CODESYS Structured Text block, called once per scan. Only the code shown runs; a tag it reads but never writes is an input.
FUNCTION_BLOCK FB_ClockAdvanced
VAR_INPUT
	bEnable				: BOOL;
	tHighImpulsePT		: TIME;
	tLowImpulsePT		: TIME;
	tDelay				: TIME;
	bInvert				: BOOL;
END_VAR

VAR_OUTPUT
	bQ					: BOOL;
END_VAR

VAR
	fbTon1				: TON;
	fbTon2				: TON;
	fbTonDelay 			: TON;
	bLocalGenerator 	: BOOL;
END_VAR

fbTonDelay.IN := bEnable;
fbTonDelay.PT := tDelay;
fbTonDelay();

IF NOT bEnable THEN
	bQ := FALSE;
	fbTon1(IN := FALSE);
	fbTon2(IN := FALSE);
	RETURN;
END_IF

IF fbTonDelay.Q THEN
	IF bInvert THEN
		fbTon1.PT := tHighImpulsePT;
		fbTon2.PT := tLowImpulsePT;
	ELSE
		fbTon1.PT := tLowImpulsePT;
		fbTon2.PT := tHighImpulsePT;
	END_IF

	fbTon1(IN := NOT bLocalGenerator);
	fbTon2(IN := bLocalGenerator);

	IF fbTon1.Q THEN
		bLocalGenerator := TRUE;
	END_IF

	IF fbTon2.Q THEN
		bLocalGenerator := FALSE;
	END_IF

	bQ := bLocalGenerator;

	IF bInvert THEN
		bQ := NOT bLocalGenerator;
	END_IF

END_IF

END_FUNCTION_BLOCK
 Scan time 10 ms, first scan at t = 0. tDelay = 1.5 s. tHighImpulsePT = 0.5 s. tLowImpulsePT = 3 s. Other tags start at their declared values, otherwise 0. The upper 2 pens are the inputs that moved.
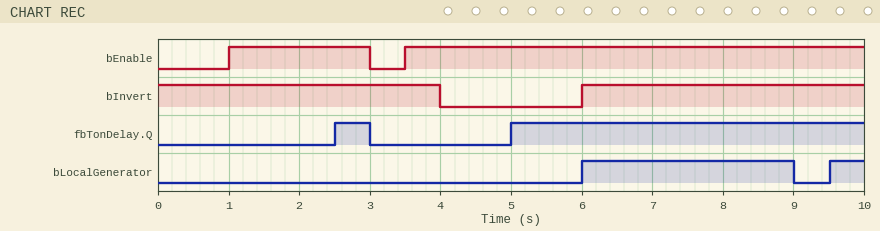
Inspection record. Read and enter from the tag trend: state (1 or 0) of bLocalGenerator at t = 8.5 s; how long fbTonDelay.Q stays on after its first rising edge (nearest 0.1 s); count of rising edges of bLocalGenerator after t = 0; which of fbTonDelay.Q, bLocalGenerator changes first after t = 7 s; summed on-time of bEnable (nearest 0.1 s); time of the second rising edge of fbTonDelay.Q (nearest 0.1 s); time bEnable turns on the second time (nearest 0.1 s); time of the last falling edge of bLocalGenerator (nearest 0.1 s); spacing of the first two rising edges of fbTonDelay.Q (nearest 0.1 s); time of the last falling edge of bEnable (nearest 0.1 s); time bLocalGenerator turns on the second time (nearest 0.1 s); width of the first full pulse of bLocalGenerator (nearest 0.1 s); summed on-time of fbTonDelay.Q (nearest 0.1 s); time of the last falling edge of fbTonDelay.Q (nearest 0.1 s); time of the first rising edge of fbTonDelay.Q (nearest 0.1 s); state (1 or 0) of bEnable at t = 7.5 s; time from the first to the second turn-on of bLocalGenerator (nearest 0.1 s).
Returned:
1
0.5 s
2
bLocalGenerator
8.5 s
5.0 s
3.5 s
9.0 s
2.5 s
3.0 s
9.5 s
3.0 s
5.5 s
3.0 s
2.5 s
1
3.5 s
